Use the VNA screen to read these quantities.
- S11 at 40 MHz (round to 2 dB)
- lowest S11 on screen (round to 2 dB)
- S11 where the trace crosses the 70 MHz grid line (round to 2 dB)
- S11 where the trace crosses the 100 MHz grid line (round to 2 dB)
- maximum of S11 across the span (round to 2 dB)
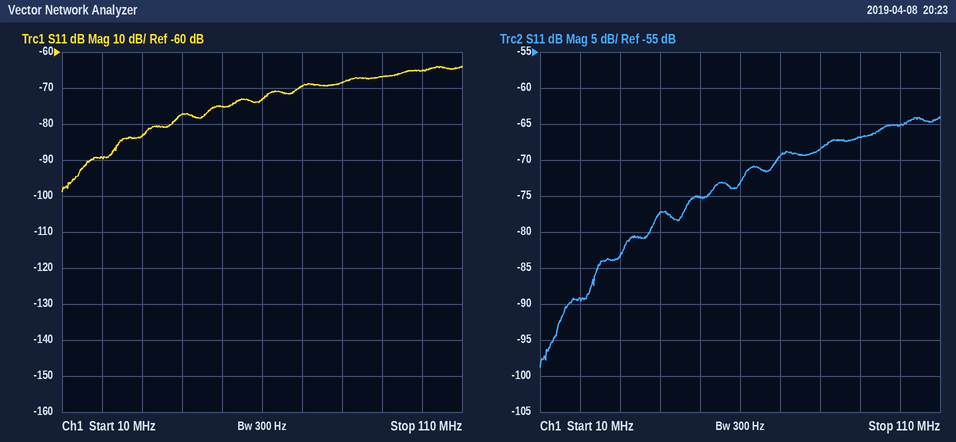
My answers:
-78 dB
-98 dB
-70 dB
-66 dB
-64 dB
